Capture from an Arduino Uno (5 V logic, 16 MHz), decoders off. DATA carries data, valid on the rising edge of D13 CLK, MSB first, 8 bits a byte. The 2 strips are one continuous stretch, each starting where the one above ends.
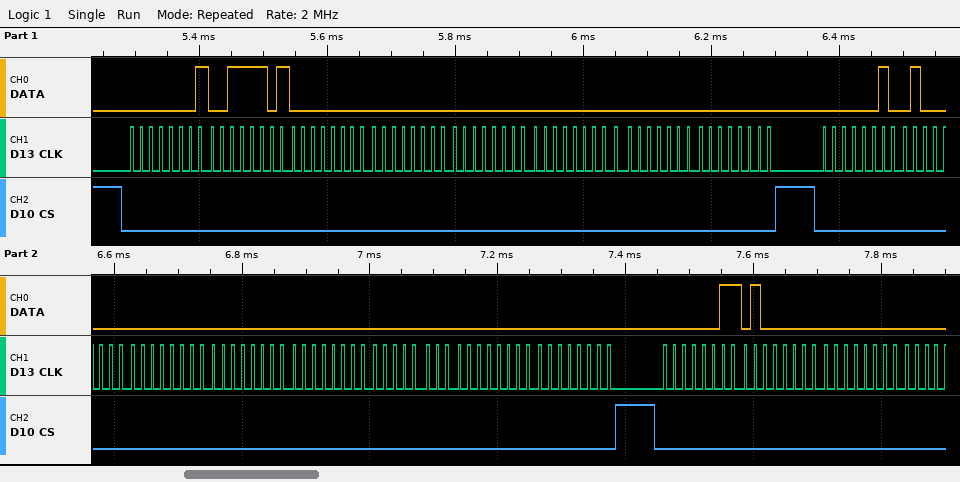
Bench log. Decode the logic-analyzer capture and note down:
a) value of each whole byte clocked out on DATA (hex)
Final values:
01 3D 00 00 00 00 00 00 02 40 00 00 00 00 00 00 03 40 00
